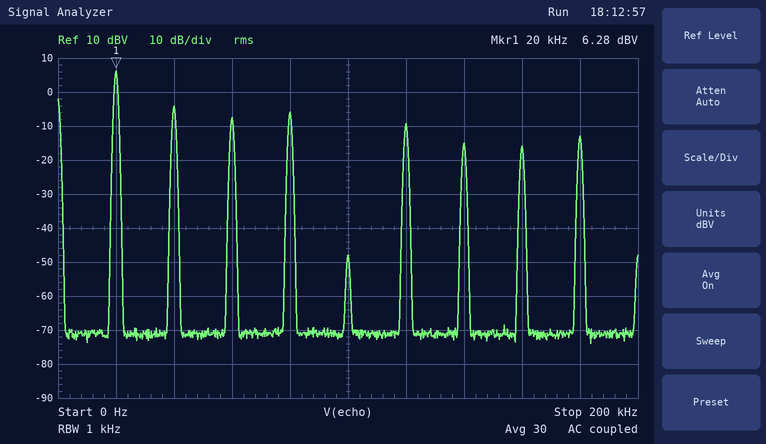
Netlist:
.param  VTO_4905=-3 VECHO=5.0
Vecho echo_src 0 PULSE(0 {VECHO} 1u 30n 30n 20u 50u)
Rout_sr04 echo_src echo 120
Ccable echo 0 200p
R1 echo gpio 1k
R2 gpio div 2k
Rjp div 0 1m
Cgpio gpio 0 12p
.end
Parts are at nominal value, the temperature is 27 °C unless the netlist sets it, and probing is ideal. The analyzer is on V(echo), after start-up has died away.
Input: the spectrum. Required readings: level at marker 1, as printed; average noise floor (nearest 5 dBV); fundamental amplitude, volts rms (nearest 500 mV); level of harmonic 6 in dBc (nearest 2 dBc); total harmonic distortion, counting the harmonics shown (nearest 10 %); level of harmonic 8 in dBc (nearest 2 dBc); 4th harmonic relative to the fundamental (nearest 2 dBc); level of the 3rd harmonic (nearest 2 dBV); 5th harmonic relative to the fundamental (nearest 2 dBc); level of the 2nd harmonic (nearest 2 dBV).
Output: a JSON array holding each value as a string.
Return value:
["6.28 dBV", "-70 dBV", "2.0 V", "-16 dBc", "50 %", "-22 dBc", "-12 dBc", "-8 dBV", "-54 dBc", "-4 dBV"]
